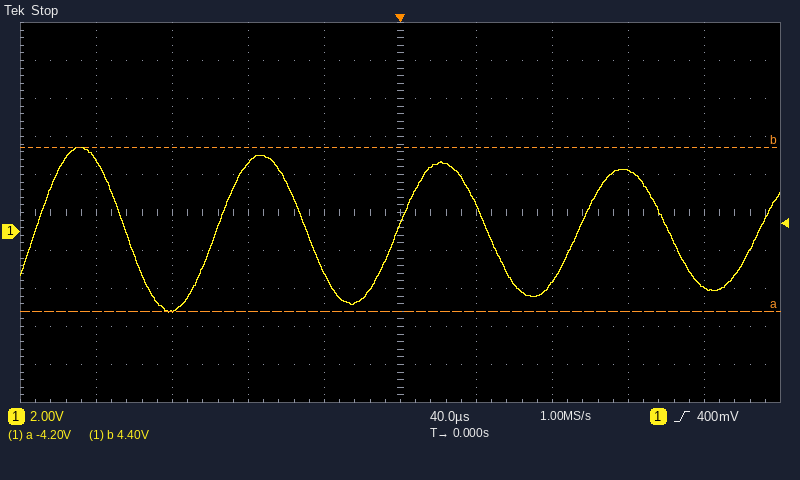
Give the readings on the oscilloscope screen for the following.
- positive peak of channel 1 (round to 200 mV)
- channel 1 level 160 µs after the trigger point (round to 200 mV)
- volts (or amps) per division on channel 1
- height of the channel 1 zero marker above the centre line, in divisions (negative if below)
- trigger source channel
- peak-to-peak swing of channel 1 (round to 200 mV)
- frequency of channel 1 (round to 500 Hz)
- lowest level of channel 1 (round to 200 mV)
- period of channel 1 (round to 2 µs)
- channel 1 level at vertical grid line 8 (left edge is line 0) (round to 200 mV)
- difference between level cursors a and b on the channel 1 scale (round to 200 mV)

4.4 V
-3.0 V
2 V
-0.5 div
channel 1
8.6 V
10.5 kHz
-4.2 V
96 µs
3.2 V
8.6 V
